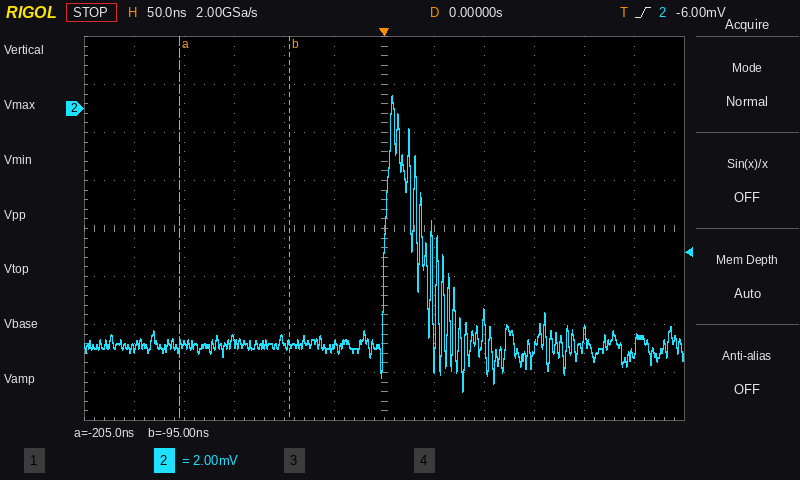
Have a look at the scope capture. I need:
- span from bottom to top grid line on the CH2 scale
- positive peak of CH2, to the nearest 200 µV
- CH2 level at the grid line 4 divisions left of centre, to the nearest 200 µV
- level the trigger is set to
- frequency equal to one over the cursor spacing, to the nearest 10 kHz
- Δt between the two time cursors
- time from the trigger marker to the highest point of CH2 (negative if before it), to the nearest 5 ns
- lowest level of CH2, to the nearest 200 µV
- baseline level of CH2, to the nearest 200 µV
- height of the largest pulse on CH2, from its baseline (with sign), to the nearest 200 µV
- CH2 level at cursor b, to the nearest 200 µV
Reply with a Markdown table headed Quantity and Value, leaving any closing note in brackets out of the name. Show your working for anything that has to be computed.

| Quantity | Value |
|---|---|
| span from bottom to top grid line on the CH2 scale | 16 mV |
| positive peak of CH2, to the nearest 200 µV | 600 µV |
| CH2 level at the grid line 4 divisions left of centre, to the nearest 200 µV | -9.8 mV |
| level the trigger is set to | -6.00 mV |
| frequency equal to one over the cursor spacing, to the nearest 10 kHz | 1 / 110 ns ≈ 9.09 MHz |
| Δt between the two time cursors | -95 ns − (-205 ns) = 110 ns |
| time from the trigger marker to the highest point of CH2 (negative if before it), to the nearest 5 ns | +10 ns |
| lowest level of CH2, to the nearest 200 µV | -11.8 mV |
| baseline level of CH2, to the nearest 200 µV | -9.8 mV |
| height of the largest pulse on CH2, from its baseline (with sign), to the nearest 200 µV | 600 µV − (-9.8 mV) = +10.4 mV |
| CH2 level at cursor b, to the nearest 200 µV | -9.8 mV |
